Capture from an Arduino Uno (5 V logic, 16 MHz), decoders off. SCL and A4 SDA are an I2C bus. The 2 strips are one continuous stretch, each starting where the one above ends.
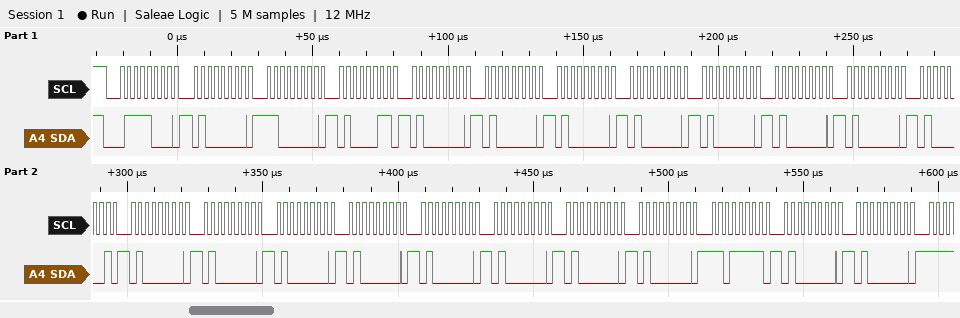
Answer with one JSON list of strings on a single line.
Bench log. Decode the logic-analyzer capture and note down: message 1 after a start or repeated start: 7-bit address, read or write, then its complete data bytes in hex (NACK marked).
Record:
["0x3C write: 40 C0 43 40 40 40 40 40 40 40 41 40 40 40 40 40 40 40 40 DF 40 40"]
